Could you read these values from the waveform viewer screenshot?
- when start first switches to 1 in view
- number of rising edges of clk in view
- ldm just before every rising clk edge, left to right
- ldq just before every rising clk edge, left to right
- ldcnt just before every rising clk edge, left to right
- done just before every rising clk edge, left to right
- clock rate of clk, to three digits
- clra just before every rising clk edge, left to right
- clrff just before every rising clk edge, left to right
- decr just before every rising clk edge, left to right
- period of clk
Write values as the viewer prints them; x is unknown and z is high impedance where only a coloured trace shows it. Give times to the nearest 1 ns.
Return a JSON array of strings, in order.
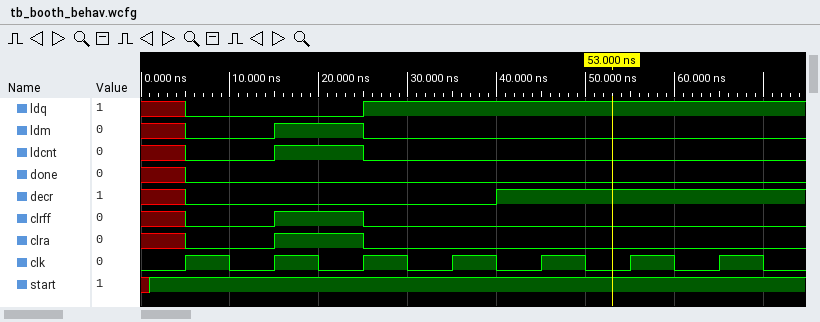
["1 ns", "7", "x 0 1 0 0 0 0", "x 0 0 1 1 1 1", "x 0 1 0 0 0 0", "x 0 0 0 0 0 0", "100 MHz", "x 0 1 0 0 0 0", "x 0 1 0 0 0 0", "x 0 0 0 1 1 1", "10 ns"]
